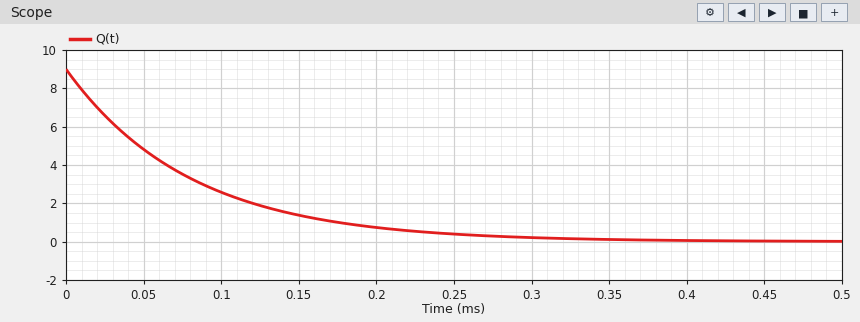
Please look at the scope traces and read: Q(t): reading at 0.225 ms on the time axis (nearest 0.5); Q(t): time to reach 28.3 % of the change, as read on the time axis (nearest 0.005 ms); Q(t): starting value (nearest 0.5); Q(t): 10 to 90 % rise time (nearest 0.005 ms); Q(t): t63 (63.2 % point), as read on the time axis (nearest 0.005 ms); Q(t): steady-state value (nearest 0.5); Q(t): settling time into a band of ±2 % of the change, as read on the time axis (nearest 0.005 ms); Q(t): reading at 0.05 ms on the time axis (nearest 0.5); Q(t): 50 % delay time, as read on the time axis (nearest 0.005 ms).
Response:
0.5
0.025 ms
9.0
0.175 ms
0.080 ms
0.0
0.315 ms
5.0
0.055 ms
